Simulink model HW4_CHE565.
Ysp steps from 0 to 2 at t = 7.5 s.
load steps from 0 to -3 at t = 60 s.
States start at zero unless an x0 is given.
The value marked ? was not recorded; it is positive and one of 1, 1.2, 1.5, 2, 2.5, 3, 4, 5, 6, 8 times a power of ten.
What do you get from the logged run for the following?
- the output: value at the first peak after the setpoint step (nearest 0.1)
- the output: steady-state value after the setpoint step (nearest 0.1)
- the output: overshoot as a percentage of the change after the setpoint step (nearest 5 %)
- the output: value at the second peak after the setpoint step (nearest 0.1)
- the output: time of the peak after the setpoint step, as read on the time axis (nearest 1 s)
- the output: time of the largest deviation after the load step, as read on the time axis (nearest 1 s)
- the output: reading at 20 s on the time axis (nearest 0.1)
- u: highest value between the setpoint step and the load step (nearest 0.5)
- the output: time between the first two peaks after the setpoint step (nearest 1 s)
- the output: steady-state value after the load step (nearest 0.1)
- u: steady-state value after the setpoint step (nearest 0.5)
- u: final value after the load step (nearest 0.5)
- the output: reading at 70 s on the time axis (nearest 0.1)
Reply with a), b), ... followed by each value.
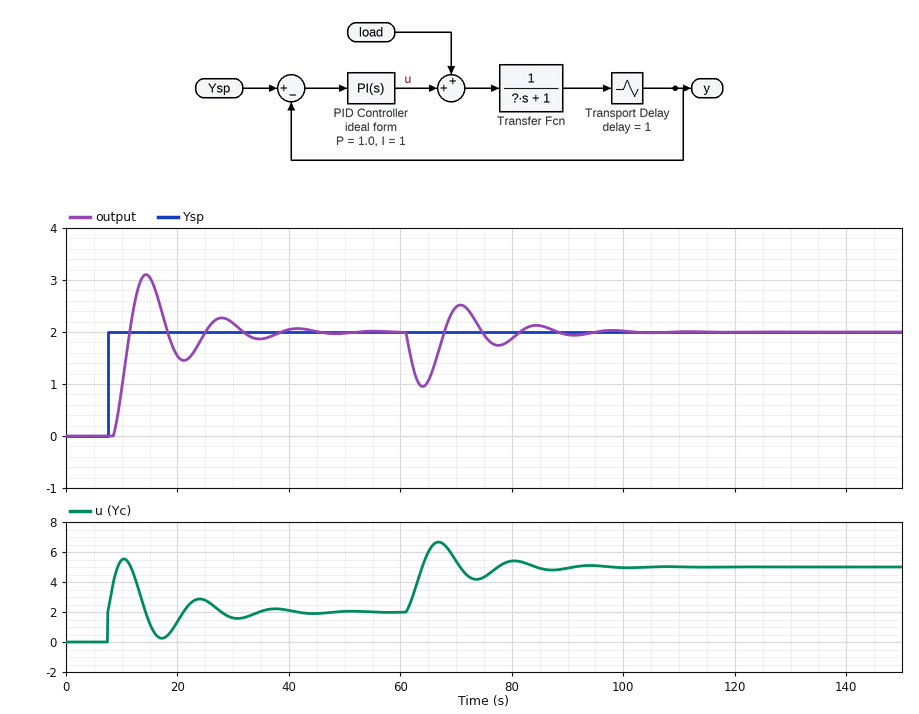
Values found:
a) 3.1
b) 2.0
c) 55 %
d) 2.3
e) 14 s
f) 64 s
g) 1.5
h) 5.5
i) 14 s
j) 2.0
k) 2.0
l) 5.0
m) 2.5
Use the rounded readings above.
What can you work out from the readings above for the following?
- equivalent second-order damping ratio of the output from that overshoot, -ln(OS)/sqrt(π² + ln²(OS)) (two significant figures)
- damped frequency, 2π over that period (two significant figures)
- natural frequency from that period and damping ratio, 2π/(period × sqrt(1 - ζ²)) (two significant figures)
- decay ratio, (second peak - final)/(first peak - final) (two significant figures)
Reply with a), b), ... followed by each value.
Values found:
a) 0.19
b) 0.45 rad/s
c) 0.46 rad/s
d) 0.27
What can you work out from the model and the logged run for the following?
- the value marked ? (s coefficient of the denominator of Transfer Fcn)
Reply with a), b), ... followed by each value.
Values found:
a) 5
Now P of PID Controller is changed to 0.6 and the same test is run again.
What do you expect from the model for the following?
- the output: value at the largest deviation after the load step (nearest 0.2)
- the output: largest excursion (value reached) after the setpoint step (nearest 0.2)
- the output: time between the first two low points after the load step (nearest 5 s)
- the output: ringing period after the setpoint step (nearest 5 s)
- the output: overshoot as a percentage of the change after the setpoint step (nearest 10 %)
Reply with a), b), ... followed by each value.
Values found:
a) 0.8
b) 2.8
c) 20 s
d) 20 s
e) 40 %
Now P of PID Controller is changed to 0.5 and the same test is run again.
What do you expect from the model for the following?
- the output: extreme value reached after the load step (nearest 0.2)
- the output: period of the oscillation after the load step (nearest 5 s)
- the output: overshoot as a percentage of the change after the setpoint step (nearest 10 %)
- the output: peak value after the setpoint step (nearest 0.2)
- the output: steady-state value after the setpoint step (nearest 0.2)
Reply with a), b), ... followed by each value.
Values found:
a) 0.8
b) 20 s
c) 40 %
d) 2.8
e) 2.0
